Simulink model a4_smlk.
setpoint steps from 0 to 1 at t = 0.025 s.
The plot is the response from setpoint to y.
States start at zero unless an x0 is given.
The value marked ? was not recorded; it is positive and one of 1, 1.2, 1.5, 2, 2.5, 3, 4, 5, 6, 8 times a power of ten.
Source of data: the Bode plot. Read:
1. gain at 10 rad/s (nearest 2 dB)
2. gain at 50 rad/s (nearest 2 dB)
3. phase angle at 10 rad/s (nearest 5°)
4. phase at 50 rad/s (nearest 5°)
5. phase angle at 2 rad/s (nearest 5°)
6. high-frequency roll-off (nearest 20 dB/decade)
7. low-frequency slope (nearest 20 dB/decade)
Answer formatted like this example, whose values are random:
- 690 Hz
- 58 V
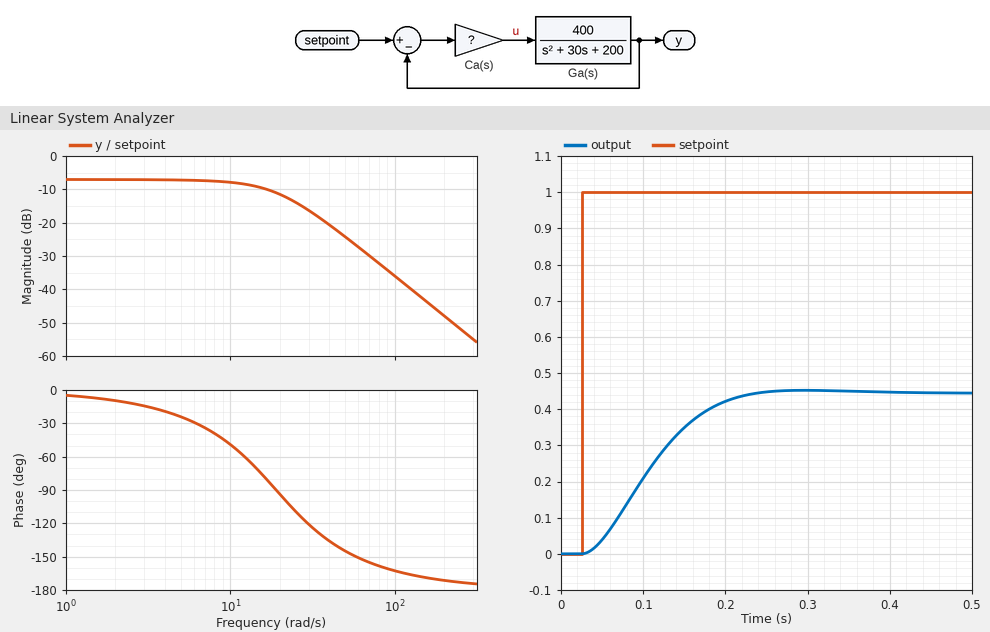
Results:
- -8 dB
- -24 dB
- -50°
- -145°
- -10°
- -40 dB/decade
- 0 dB/decade
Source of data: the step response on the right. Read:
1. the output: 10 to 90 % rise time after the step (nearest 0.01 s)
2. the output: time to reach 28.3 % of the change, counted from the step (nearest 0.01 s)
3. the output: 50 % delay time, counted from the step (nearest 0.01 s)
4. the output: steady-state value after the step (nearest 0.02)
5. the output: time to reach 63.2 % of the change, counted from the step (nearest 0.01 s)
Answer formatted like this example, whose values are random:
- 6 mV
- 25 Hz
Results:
- 0.13 s
- 0.05 s
- 0.08 s
- 0.44
- 0.10 s
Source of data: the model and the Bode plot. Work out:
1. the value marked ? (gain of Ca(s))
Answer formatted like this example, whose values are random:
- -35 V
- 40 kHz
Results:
- 0.4
